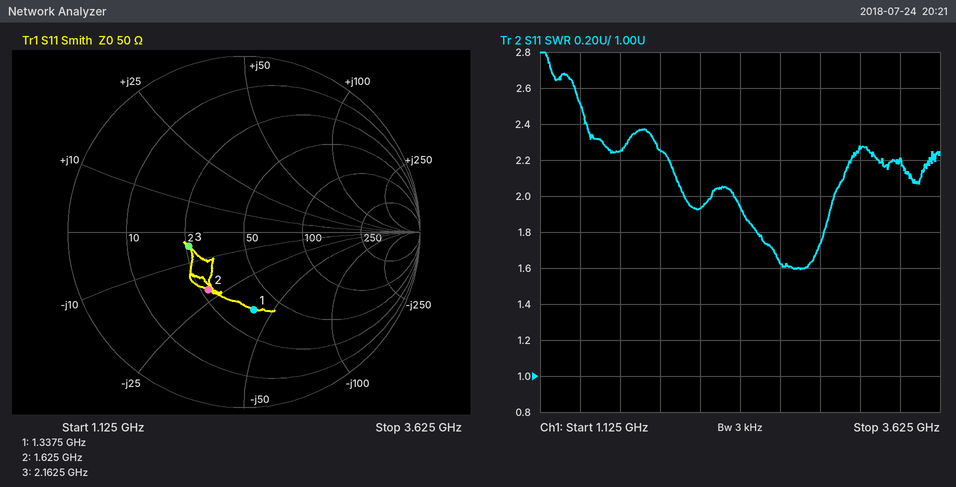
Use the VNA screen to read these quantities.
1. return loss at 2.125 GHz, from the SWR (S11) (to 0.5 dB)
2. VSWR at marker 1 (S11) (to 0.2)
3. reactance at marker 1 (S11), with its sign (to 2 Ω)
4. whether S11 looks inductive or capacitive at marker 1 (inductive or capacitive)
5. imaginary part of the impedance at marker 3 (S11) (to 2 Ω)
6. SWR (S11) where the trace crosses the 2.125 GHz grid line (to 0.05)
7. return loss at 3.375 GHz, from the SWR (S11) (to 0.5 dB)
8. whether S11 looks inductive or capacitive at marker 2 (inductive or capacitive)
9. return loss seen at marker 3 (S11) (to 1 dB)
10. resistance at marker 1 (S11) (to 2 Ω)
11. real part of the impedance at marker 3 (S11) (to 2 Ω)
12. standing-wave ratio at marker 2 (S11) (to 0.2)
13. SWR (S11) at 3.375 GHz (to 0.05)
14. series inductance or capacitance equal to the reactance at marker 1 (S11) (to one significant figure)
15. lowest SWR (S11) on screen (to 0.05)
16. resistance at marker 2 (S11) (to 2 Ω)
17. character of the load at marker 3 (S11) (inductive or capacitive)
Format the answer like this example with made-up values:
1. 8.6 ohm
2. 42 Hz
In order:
1. 10.0 dB
2. 2.6
3. -40 Ω
4. capacitive
5. -4 Ω
6. 1.95
7. 8.5 dB
8. capacitive
9. 10 dB
10. 36 Ω
11. 26 Ω
12. 2.2
13. 2.20
14. 3 pF
15. 1.60
16. 28 Ω
17. capacitive
